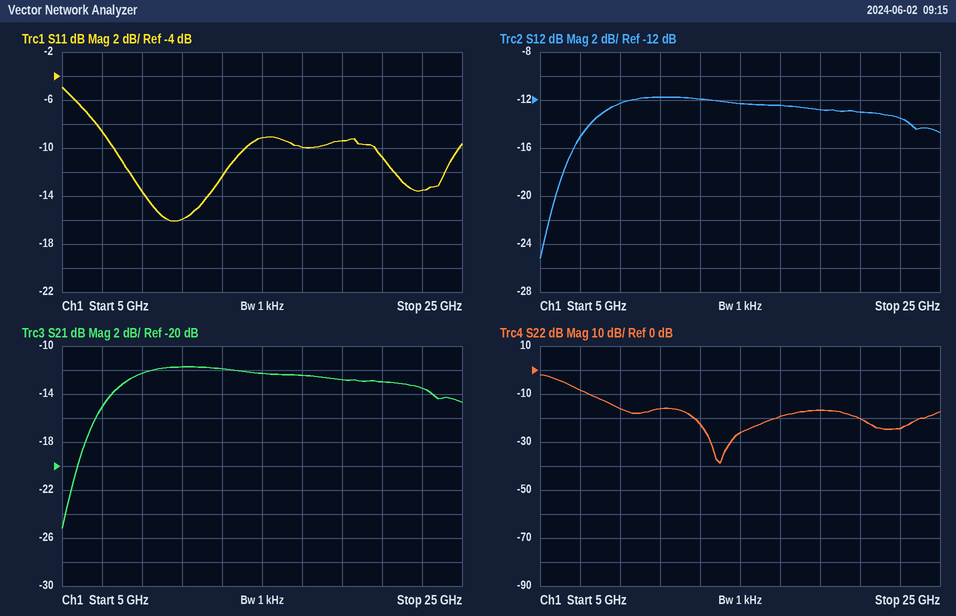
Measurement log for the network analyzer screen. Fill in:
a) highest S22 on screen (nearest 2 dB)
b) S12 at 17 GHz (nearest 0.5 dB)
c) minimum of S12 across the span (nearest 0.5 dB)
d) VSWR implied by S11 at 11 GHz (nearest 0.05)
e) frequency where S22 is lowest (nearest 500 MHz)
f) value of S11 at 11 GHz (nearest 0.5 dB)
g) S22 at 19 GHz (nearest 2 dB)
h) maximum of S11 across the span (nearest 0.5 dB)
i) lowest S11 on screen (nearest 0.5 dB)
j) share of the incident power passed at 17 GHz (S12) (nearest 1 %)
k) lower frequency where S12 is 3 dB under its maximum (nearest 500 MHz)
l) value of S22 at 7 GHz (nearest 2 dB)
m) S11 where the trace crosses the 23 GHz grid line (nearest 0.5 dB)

-2 dB
-12.5 dB
-25.0 dB
1.40
14.0 GHz
-16.0 dB
-16 dB
-5.0 dB
-16.0 dB
6 %
7.0 GHz
-8 dB
-13.5 dB
